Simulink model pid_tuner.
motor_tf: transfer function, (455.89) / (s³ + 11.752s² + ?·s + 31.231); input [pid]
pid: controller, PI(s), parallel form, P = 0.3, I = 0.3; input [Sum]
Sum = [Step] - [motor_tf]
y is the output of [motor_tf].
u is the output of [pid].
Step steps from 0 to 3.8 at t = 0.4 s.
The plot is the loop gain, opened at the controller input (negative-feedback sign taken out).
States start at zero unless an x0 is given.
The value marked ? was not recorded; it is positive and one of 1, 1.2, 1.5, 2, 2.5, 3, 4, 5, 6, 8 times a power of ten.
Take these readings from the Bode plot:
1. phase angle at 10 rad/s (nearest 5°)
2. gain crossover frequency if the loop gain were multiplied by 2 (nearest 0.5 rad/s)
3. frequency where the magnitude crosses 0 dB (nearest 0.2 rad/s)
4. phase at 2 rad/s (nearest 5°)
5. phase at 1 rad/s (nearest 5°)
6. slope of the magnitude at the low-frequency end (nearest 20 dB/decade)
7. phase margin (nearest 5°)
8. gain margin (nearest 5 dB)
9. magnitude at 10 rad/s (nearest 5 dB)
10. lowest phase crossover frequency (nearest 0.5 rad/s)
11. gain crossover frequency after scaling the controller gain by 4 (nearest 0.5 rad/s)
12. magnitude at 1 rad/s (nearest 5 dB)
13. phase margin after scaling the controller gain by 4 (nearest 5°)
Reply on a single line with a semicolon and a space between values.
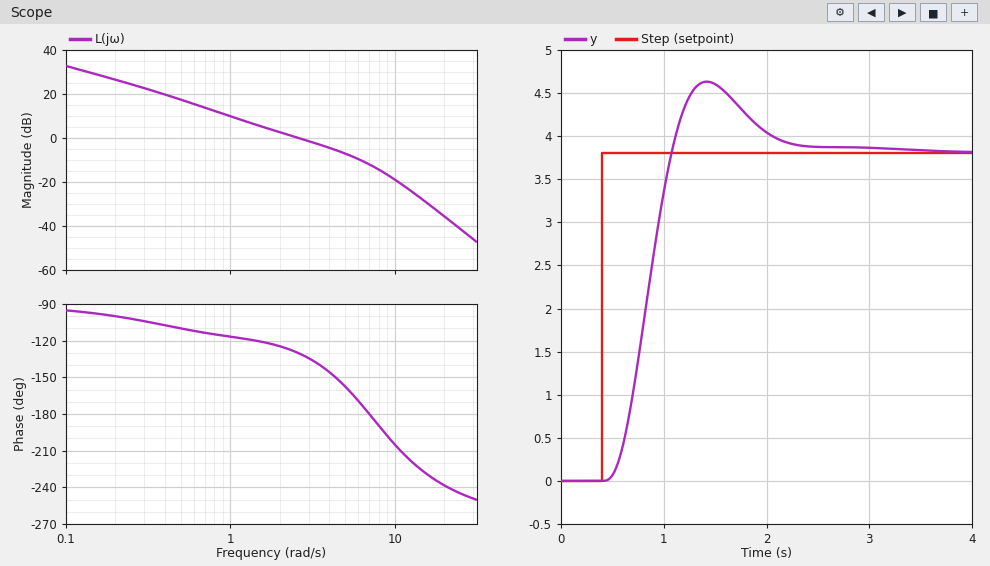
-205°; 4.5 rad/s; 2.6 rad/s; -125°; -115°; -20 dB/decade; 50°; 10 dB; -20 dB; 7.0 rad/s; 7.0 rad/s; 10 dB; 0°
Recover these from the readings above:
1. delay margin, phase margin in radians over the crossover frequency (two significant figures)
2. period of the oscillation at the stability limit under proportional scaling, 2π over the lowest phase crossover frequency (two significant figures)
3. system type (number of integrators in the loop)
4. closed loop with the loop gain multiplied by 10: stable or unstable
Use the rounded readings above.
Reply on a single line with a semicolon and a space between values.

0.34 s; 0.90 s; 1; unstable
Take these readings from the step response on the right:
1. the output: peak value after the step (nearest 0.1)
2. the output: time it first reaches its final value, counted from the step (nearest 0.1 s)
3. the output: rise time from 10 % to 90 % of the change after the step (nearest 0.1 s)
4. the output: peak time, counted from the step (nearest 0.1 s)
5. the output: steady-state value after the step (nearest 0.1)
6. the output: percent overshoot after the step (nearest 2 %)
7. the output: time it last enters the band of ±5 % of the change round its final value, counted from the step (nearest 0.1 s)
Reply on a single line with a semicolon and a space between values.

4.6; 0.7 s; 0.4 s; 1.0 s; 3.8; 22 %; 1.7 s
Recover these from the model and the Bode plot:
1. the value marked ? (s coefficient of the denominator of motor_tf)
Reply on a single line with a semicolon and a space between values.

60
